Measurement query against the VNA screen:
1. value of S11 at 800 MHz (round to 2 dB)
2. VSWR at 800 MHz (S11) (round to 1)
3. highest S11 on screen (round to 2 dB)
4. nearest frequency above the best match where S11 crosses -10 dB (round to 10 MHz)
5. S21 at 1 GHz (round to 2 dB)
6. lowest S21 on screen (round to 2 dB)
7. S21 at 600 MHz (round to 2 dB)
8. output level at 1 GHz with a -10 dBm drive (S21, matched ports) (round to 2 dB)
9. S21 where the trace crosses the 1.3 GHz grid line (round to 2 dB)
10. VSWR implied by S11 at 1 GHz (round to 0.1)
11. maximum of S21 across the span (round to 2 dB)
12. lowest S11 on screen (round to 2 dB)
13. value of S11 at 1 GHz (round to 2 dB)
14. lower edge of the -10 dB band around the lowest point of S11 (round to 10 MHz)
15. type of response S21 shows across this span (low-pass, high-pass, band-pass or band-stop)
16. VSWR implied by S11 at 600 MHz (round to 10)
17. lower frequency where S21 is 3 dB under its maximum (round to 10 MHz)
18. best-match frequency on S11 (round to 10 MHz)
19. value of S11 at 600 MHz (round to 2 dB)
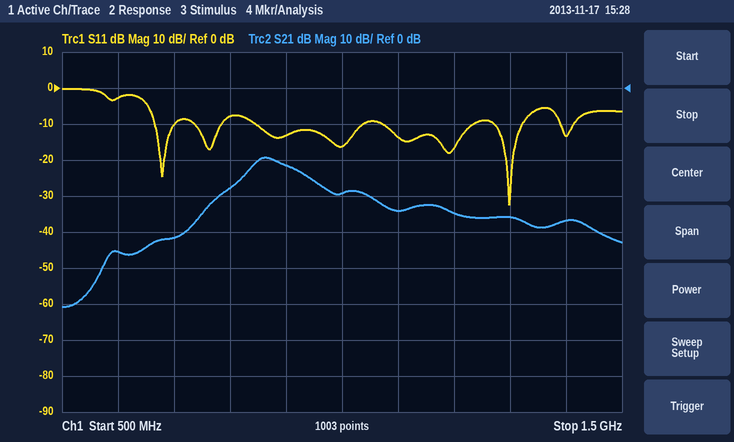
-8 dB
2
0 dB
1.32 GHz
-30 dB
-60 dB
-46 dB
-40 dBm
-36 dB
1.4
-20 dB
-32 dB
-16 dB
1.27 GHz
band-pass
10
840 MHz
1.30 GHz
-2 dB
